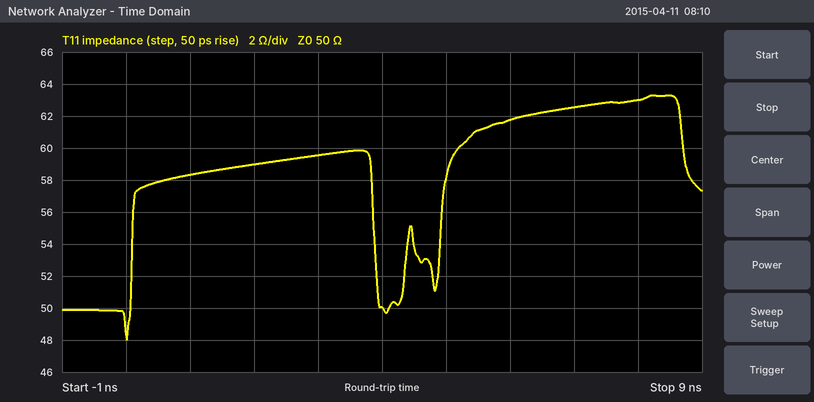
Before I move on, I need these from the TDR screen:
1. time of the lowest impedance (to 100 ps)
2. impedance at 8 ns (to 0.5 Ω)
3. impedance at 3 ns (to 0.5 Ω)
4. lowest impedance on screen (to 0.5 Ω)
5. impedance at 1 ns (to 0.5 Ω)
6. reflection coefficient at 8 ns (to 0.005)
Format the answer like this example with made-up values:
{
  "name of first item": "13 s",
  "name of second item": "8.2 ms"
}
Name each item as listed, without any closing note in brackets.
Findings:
{
  "time of the lowest impedance": "0.0 ns",
  "impedance at 8 ns": "63.0 Ω",
  "impedance at 3 ns": "59.5 Ω",
  "lowest impedance on screen": "48.0 Ω",
  "impedance at 1 ns": "58.5 Ω",
  "reflection coefficient at 8 ns": "+0.115"
}
